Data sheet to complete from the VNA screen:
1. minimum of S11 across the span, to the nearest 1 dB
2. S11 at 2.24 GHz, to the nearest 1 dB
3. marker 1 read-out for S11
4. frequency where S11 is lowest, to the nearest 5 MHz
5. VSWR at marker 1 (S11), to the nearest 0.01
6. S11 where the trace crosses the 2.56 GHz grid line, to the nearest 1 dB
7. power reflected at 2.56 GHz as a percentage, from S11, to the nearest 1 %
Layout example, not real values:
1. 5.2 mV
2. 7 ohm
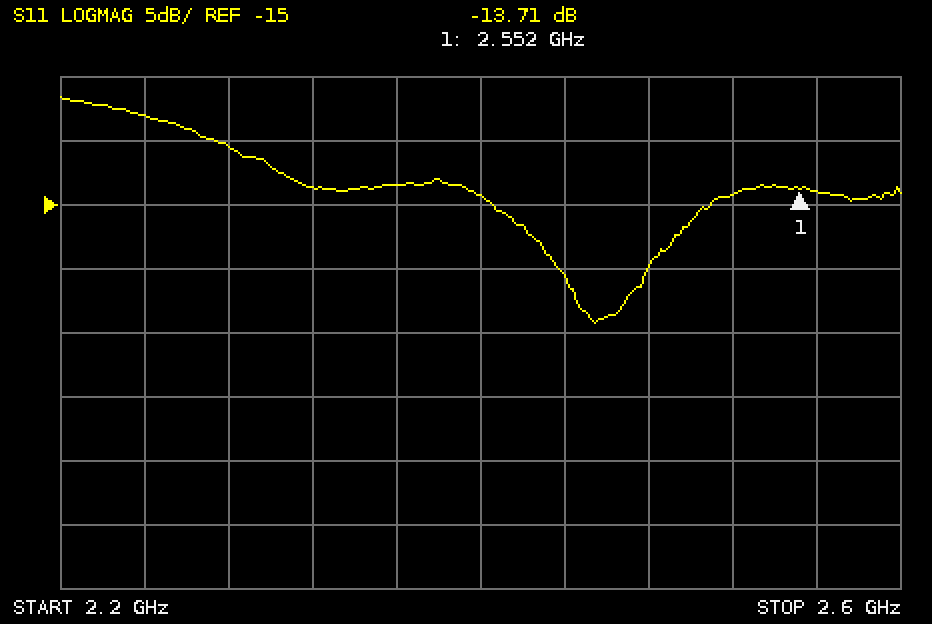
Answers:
1. -24 dB
2. -8 dB
3. -13.71 dB
4. 2.455 GHz
5. 1.52
6. -14 dB
7. 4 %
